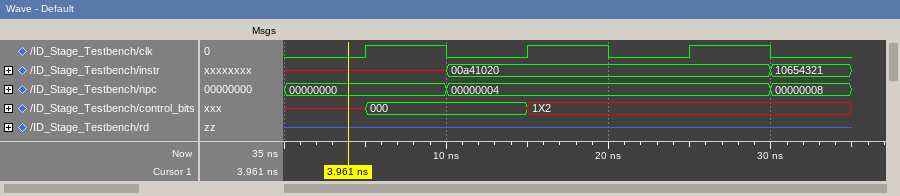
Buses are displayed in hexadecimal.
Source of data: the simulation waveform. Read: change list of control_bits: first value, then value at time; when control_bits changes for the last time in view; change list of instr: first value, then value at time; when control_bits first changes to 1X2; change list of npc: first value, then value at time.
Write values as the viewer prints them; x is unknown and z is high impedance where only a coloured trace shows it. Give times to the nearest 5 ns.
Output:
x, 000 at 5 ns, 1X2 at 15 ns
15 ns
x, 00a41020 at 10 ns, 10654321 at 30 ns
15 ns
00000000, 00000004 at 10 ns, 00000008 at 30 ns
